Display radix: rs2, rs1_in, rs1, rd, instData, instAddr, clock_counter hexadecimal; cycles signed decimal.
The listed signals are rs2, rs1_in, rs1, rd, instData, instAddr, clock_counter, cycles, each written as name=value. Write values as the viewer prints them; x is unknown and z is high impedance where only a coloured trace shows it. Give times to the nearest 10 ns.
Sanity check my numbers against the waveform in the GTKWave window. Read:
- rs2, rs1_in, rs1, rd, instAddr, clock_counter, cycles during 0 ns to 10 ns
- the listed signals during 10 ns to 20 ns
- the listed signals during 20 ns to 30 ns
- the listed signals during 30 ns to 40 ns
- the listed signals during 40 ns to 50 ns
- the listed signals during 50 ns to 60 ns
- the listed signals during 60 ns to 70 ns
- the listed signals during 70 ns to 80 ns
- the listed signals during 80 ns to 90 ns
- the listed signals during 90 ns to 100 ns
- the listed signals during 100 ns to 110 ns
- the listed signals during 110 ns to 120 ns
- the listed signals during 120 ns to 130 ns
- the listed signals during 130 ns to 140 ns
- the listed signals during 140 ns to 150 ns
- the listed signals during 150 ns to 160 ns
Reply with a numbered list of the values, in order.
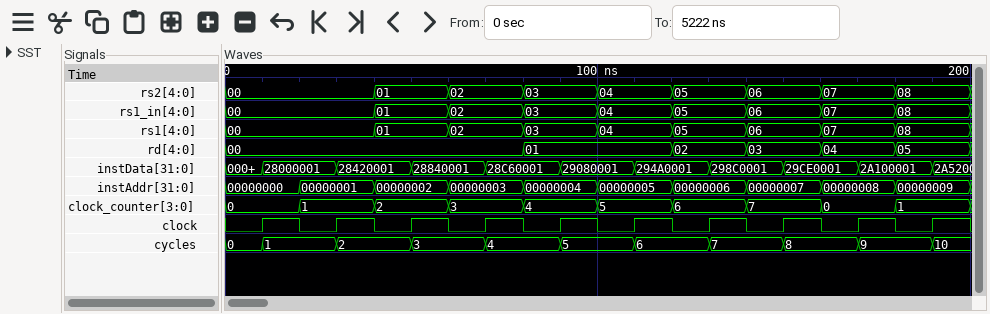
1. rs2=00, rs1_in=00, rs1=00, rd=00, instAddr=00000000, clock_counter=0, cycles=0
2. rs2=00, rs1_in=00, rs1=00, rd=00, instData=28000001, instAddr=00000000, clock_counter=0, cycles=1
3. rs2=00, rs1_in=00, rs1=00, rd=00, instData=28000001, instAddr=00000001, clock_counter=1, cycles=1
4. rs2=00, rs1_in=00, rs1=00, rd=00, instData=28420001, instAddr=00000001, clock_counter=1, cycles=2
5. rs2=01, rs1_in=01, rs1=01, rd=00, instData=28420001, instAddr=00000002, clock_counter=2, cycles=2
6. rs2=01, rs1_in=01, rs1=01, rd=00, instData=28840001, instAddr=00000002, clock_counter=2, cycles=3
7. rs2=02, rs1_in=02, rs1=02, rd=00, instData=28840001, instAddr=00000003, clock_counter=3, cycles=3
8. rs2=02, rs1_in=02, rs1=02, rd=00, instData=28C60001, instAddr=00000003, clock_counter=3, cycles=4
9. rs2=03, rs1_in=03, rs1=03, rd=01, instData=28C60001, instAddr=00000004, clock_counter=4, cycles=4
10. rs2=03, rs1_in=03, rs1=03, rd=01, instData=29080001, instAddr=00000004, clock_counter=4, cycles=5
11. rs2=04, rs1_in=04, rs1=04, rd=01, instData=29080001, instAddr=00000005, clock_counter=5, cycles=5
12. rs2=04, rs1_in=04, rs1=04, rd=01, instData=294A0001, instAddr=00000005, clock_counter=5, cycles=6
13. rs2=05, rs1_in=05, rs1=05, rd=02, instData=294A0001, instAddr=00000006, clock_counter=6, cycles=6
14. rs2=05, rs1_in=05, rs1=05, rd=02, instData=298C0001, instAddr=00000006, clock_counter=6, cycles=7
15. rs2=06, rs1_in=06, rs1=06, rd=03, instData=298C0001, instAddr=00000007, clock_counter=7, cycles=7
16. rs2=06, rs1_in=06, rs1=06, rd=03, instData=29CE0001, instAddr=00000007, clock_counter=7, cycles=8
